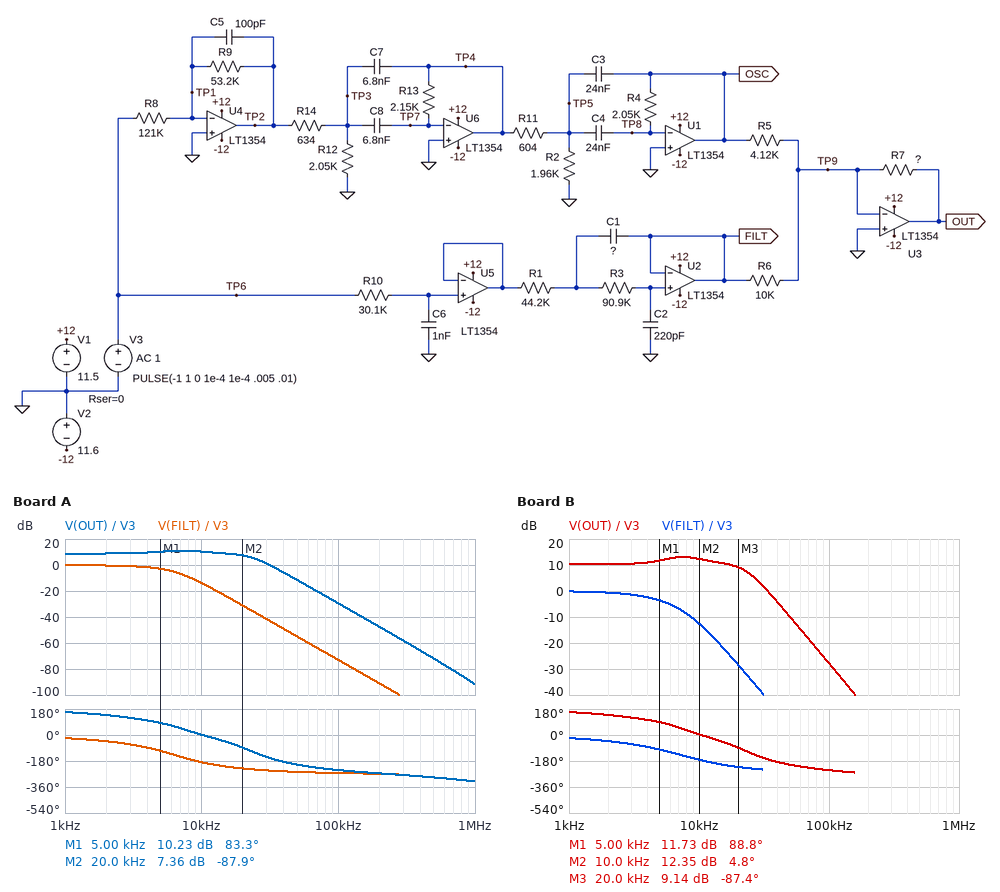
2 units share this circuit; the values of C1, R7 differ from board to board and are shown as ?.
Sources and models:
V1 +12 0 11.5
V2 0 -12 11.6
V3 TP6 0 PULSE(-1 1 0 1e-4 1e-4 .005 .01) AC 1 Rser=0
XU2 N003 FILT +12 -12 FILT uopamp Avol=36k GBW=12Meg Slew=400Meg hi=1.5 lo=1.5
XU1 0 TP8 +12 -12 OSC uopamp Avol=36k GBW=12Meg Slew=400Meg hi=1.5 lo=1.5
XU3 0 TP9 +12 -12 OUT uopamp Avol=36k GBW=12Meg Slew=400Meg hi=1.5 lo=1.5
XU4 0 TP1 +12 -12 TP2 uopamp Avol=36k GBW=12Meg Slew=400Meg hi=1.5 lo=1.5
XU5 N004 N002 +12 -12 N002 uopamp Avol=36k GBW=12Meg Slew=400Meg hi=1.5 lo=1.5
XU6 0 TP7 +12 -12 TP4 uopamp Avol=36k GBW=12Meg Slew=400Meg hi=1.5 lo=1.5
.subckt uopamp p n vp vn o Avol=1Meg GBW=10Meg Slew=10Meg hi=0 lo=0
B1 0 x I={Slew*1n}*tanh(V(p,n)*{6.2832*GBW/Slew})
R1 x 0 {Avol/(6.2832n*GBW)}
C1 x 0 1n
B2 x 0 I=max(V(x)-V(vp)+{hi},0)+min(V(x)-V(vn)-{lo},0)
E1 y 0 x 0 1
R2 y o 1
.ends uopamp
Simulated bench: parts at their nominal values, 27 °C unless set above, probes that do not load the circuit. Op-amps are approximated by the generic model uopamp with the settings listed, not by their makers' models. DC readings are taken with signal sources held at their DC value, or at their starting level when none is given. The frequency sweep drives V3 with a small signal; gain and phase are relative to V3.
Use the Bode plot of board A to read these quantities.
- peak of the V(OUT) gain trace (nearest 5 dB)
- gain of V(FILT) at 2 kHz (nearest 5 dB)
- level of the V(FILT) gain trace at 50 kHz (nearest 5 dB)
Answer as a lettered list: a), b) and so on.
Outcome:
a) 10 dB
b) 0 dB
c) -55 dB
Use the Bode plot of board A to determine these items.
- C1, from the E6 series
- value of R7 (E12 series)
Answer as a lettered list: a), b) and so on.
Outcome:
a) 680 pF
b) 27 kΩ
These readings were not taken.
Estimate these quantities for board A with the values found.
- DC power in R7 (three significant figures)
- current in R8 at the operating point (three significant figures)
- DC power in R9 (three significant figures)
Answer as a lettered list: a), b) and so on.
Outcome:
a) 270 µW
b) 8.26 µA
c) 3.63 µW
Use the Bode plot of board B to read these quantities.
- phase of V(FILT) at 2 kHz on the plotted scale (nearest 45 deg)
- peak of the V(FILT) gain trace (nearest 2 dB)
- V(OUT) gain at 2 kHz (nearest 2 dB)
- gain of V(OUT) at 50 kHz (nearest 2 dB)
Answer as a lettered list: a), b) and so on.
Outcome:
a) -45 deg
b) 0 dB
c) 10 dB
d) -10 dB
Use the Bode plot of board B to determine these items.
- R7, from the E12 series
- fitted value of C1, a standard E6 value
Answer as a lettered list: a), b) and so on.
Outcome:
a) 33 kΩ
b) 470 pF
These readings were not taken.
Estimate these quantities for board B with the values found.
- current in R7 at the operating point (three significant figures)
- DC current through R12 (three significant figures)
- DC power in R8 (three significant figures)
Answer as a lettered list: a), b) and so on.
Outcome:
a) 100 µA
b) 164 µA
c) 8.26 µW
